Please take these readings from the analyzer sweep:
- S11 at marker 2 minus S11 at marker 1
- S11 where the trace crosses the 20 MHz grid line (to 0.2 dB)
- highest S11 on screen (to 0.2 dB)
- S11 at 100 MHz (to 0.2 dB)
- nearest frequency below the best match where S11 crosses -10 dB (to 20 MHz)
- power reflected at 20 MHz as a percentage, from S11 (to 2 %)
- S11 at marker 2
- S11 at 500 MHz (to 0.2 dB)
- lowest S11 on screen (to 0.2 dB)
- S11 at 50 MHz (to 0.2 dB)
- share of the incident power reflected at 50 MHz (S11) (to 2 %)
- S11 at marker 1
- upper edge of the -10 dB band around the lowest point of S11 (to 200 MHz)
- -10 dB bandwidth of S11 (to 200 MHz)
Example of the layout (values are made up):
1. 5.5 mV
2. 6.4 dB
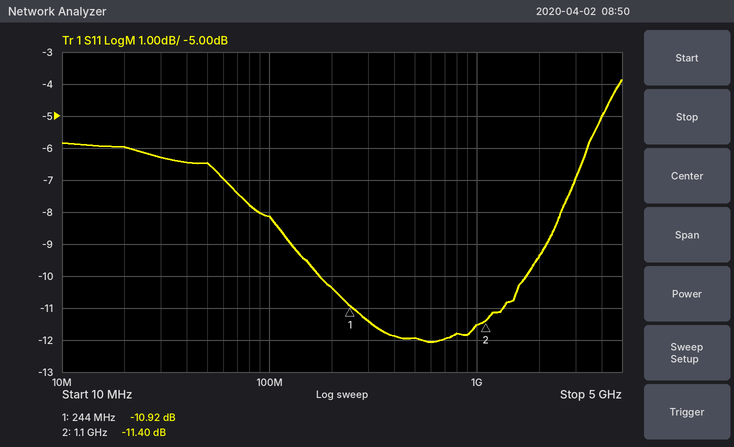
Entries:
1. -0.48 dB
2. -6.0 dB
3. -3.8 dB
4. -8.2 dB
5. 180 MHz
6. 26 %
7. -11.40 dB
8. -12.0 dB
9. -12.0 dB
10. -6.4 dB
11. 22 %
12. -10.92 dB
13. 1.8 GHz
14. 1.6 GHz
